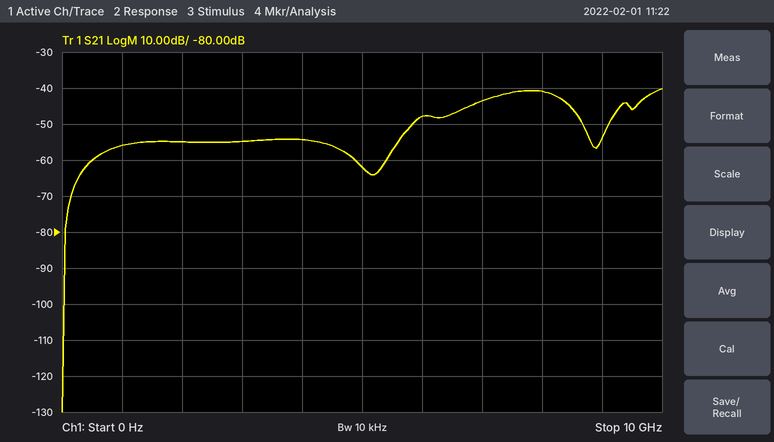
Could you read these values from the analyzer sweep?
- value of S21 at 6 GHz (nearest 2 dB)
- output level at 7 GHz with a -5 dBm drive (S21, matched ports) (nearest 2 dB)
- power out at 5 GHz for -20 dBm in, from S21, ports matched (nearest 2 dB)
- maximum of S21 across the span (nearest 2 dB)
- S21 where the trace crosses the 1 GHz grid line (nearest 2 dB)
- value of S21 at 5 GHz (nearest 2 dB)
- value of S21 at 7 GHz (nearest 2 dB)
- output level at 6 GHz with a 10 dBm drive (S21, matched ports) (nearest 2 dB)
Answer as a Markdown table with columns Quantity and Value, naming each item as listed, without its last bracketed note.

| Quantity | Value |
|---|---|
| value of S21 at 6 GHz | -48 dB |
| output level at 7 GHz with a -5 dBm drive (S21, matched ports) | -48 dBm |
| power out at 5 GHz for -20 dBm in, from S21, ports matched | -82 dBm |
| maximum of S21 across the span | -40 dB |
| S21 where the trace crosses the 1 GHz grid line | -56 dB |
| value of S21 at 5 GHz | -62 dB |
| value of S21 at 7 GHz | -44 dB |
| output level at 6 GHz with a 10 dBm drive (S21, matched ports) | -38 dBm |
